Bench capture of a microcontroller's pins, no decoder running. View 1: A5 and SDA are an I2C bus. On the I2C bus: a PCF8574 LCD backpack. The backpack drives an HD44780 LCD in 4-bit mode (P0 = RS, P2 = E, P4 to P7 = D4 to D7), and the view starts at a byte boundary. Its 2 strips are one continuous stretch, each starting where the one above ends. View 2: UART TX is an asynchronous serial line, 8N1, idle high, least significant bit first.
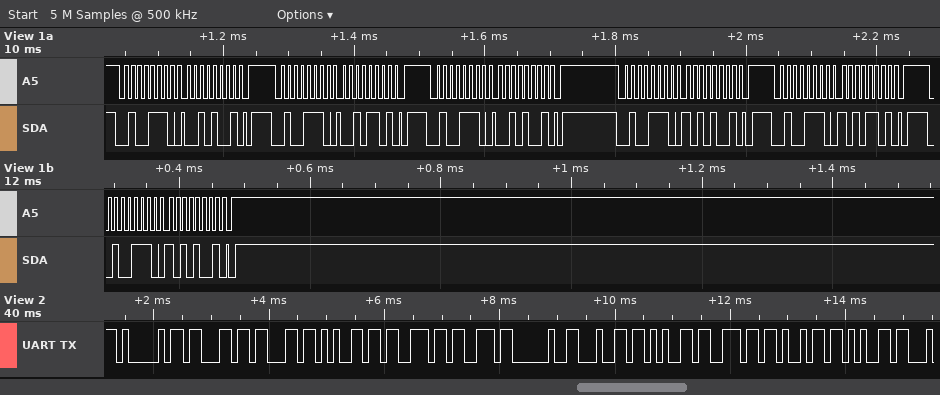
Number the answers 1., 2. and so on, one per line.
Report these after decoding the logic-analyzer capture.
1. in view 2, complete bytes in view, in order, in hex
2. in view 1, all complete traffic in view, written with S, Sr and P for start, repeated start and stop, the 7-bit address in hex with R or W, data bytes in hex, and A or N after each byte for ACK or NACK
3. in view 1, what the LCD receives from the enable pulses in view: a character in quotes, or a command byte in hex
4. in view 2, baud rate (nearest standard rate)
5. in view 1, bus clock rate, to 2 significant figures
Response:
1. 41 63 63 65 73 73 20 64 65 6E 69 65
2. S 27W A 29 A P S 27W A 2D A P S 27W A 29 A P S 27W A A9 A P S 27W A AD A P S 27W A A9 A P
3. '*'
4. 9600 baud
5. 100 kHz
